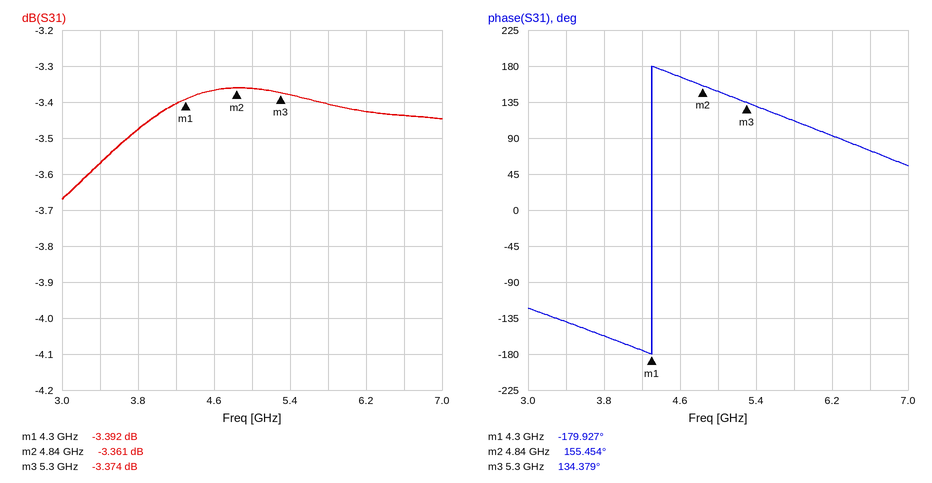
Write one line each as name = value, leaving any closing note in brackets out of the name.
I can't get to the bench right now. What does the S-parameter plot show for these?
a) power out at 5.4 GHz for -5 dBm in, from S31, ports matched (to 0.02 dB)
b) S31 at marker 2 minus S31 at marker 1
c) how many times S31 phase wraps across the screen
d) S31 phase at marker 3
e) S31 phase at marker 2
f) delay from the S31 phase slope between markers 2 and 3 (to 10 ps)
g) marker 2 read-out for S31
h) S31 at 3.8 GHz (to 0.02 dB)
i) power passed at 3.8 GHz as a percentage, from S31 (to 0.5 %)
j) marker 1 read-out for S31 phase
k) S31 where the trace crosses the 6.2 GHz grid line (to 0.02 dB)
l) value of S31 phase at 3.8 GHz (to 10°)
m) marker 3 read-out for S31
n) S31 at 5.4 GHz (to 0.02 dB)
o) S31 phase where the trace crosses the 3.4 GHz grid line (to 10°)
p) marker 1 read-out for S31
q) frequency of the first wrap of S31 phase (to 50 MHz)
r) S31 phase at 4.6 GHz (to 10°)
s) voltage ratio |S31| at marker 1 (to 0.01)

power out at 5.4 GHz for -5 dBm in, from S31, ports matched = -8.38 dBm
S31 at marker 2 minus S31 at marker 1 = 0.031 dB
how many times S31 phase wraps across the screen = 1
S31 phase at marker 3 = 134.379°
S31 phase at marker 2 = 155.454°
delay from the S31 phase slope between markers 2 and 3 = 130 ps
marker 2 read-out for S31 = -3.361 dB
S31 at 3.8 GHz = -3.48 dB
power passed at 3.8 GHz as a percentage, from S31 = 45.0 %
marker 1 read-out for S31 phase = -179.927°
S31 where the trace crosses the 6.2 GHz grid line = -3.42 dB
value of S31 phase at 3.8 GHz = -160°
marker 3 read-out for S31 = -3.374 dB
S31 at 5.4 GHz = -3.38 dB
S31 phase where the trace crosses the 3.4 GHz grid line = -140°
marker 1 read-out for S31 = -3.392 dB
frequency of the first wrap of S31 phase = 4.30 GHz
S31 phase at 4.6 GHz = 170°
voltage ratio |S31| at marker 1 = 0.68
